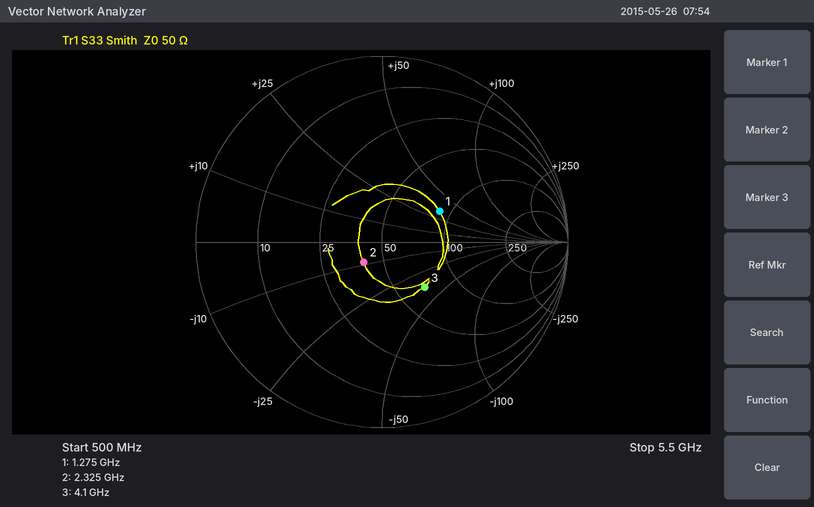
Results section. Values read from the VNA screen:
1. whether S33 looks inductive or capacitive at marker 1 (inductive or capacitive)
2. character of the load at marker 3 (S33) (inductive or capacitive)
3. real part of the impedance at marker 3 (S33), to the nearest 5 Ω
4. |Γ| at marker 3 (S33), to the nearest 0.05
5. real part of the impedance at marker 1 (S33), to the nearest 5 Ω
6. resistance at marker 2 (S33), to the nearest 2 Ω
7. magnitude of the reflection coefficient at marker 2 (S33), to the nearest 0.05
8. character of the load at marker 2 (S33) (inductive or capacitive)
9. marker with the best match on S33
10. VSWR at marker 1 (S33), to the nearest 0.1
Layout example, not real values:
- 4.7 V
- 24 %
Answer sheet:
- inductive
- capacitive
- 70 Ω
- 0.35
- 85 Ω
- 40 Ω
- 0.15
- capacitive
- marker 2
- 2.1
